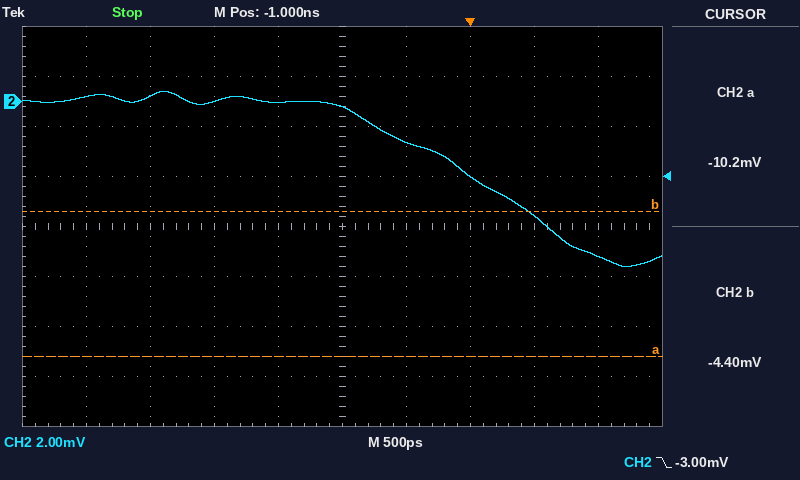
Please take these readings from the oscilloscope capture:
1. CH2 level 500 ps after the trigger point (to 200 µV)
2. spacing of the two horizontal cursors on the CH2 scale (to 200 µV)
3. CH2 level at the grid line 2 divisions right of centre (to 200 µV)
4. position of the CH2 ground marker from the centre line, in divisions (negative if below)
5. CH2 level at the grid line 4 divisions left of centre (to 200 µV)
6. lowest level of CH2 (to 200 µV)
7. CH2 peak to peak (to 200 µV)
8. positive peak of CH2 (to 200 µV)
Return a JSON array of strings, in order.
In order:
["-4.6 mV", "5.8 mV", "-3.0 mV", "+2.5 div", "200 µV", "-6.6 mV", "7.0 mV", "400 µV"]
